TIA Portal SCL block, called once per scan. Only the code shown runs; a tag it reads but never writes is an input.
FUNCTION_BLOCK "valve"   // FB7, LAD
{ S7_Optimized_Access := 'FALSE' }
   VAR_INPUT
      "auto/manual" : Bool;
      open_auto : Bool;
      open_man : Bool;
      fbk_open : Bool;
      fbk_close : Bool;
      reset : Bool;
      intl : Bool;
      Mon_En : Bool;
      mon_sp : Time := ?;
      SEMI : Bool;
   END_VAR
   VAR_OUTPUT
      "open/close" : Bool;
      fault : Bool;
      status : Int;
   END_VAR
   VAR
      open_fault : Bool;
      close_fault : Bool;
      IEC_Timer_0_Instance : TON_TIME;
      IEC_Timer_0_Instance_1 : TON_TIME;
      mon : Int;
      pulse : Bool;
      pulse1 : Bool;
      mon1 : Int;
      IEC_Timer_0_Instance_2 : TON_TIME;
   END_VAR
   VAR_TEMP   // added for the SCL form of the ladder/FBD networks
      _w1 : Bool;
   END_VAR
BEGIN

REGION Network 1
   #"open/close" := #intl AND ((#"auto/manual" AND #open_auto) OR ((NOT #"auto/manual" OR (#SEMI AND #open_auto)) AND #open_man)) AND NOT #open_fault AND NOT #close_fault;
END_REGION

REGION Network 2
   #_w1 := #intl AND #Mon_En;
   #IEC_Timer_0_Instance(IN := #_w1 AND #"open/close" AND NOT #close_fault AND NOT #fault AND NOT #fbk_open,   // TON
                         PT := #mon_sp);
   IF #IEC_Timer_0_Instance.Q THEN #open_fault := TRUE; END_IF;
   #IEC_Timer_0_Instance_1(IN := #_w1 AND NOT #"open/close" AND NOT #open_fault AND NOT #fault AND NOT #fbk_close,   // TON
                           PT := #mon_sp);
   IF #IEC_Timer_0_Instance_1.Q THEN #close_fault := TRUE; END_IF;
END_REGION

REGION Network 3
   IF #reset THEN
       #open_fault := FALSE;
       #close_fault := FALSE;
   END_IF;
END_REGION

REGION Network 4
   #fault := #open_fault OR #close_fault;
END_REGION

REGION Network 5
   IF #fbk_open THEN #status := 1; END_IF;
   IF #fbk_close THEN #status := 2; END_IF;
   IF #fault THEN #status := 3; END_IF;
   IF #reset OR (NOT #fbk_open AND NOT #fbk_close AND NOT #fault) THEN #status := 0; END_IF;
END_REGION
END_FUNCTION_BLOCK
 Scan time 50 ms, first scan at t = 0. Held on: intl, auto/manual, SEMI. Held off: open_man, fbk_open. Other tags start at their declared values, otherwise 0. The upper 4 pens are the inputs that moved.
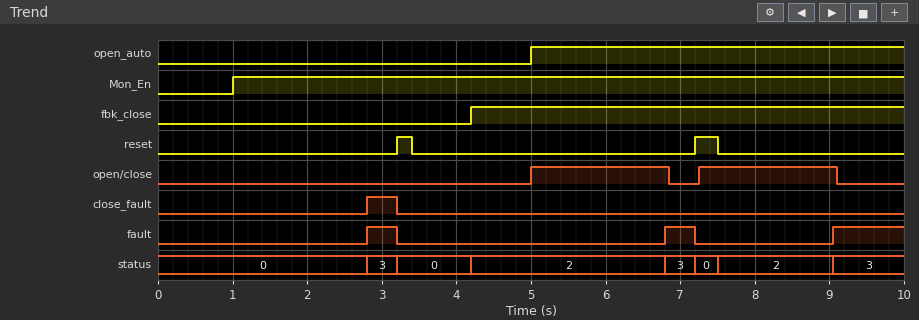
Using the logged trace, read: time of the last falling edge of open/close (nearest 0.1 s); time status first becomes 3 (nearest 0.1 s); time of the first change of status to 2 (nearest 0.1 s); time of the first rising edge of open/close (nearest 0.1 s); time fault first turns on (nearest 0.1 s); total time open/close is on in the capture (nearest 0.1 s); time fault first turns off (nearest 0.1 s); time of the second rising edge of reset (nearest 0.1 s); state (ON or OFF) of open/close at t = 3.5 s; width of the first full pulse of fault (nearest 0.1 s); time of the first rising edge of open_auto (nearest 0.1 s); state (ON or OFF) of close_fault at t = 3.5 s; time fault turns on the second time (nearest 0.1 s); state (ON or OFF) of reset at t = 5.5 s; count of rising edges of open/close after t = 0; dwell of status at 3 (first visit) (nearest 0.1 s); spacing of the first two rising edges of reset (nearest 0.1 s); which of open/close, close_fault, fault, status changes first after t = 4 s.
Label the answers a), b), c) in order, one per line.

a) 9.1 s
b) 2.8 s
c) 4.2 s
d) 5.0 s
e) 2.8 s
f) 3.7 s
g) 3.2 s
h) 7.2 s
i) OFF
j) 0.4 s
k) 5.0 s
l) OFF
m) 6.8 s
n) OFF
o) 2
p) 0.4 s
q) 4.0 s
r) status
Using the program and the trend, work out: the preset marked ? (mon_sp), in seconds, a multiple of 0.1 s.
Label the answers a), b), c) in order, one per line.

a) 1.8 s
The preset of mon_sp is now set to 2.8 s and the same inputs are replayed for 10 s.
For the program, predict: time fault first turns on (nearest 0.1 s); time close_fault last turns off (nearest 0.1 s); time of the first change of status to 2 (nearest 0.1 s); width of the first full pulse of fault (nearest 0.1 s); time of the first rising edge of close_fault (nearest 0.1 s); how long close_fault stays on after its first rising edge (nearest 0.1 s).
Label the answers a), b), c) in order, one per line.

a) 3.8 s
b) 7.2 s
c) 7.5 s
d) 3.4 s
e) 3.8 s
f) 3.4 s
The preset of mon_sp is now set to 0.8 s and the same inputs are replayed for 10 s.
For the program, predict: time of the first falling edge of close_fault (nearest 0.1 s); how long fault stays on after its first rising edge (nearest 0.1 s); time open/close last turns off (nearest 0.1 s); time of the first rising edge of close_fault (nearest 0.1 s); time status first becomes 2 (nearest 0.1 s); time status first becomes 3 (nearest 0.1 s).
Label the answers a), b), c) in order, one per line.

a) 3.2 s
b) 1.4 s
c) 8.1 s
d) 1.8 s
e) 7.5 s
f) 1.8 s
